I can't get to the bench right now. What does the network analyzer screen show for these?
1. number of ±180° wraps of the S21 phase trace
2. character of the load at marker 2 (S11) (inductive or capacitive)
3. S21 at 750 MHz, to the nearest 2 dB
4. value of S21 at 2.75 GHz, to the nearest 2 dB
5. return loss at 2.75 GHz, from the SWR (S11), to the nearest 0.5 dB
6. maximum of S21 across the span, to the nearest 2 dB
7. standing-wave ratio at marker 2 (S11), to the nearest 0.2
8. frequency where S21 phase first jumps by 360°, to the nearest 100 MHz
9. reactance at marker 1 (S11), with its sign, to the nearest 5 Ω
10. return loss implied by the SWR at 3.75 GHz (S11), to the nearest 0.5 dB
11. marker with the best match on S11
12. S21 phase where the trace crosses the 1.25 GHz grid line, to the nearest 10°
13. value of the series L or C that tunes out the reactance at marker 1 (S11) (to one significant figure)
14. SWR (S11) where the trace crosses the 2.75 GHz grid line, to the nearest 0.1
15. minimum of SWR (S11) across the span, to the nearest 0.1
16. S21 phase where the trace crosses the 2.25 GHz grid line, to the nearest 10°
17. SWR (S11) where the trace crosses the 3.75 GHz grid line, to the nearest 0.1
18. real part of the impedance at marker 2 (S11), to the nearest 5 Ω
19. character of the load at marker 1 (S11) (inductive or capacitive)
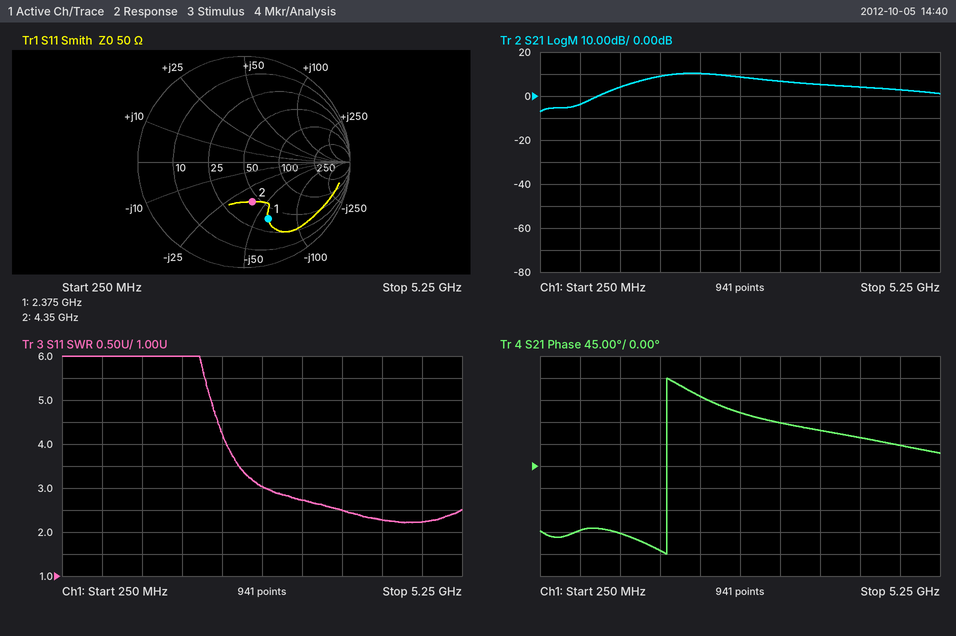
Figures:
1
capacitive
-4 dB
8 dB
6.0 dB
10 dB
2.2
1.8 GHz
-60 Ω
7.5 dB
marker 2
-140°
4 nH
3.0
2.2
140°
2.5
45 Ω
capacitive
